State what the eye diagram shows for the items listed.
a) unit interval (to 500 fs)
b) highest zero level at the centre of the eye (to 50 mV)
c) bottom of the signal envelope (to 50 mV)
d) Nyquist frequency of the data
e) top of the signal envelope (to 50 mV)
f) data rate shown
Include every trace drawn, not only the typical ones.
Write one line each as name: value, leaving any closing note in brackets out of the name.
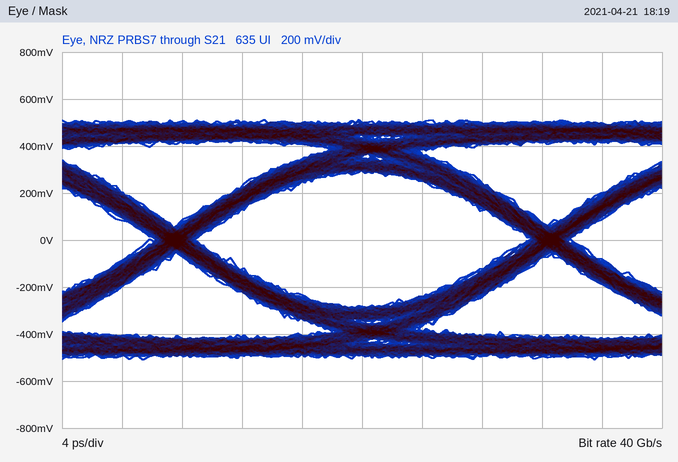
unit interval: 25.0 ps
highest zero level at the centre of the eye: -300 mV
bottom of the signal envelope: -500 mV
Nyquist frequency of the data: 20 GHz
top of the signal envelope: 500 mV
data rate shown: 40 Gb/s
